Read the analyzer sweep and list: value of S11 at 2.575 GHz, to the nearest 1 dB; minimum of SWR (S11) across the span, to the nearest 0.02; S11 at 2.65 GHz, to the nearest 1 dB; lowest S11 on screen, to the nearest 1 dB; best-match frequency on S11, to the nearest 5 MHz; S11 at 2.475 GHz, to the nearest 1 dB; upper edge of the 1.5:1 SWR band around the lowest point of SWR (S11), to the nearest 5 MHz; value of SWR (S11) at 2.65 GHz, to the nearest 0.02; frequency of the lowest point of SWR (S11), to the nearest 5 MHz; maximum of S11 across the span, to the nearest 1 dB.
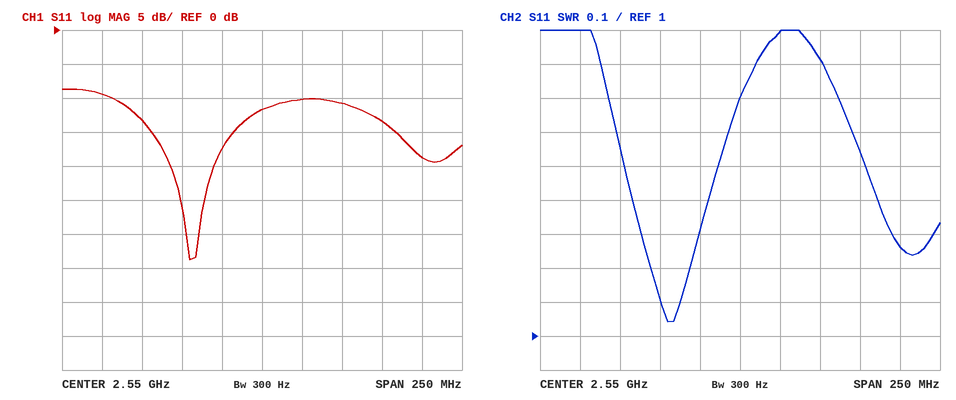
-10 dB
1.04
-19 dB
-34 dB
2.505 GHz
-13 dB
2.535 GHz
1.26
2.505 GHz
-9 dB
